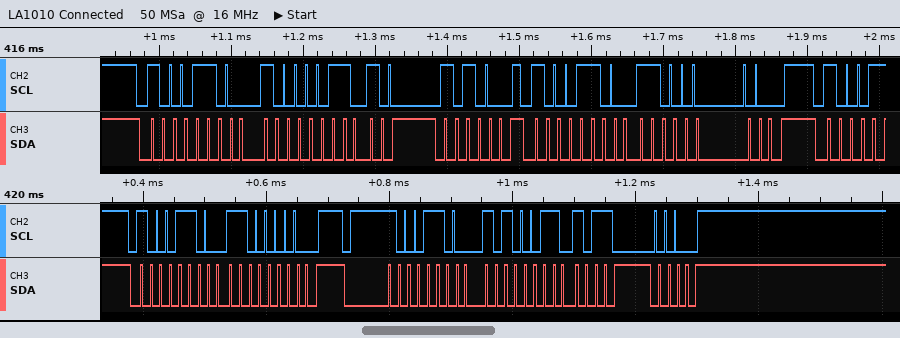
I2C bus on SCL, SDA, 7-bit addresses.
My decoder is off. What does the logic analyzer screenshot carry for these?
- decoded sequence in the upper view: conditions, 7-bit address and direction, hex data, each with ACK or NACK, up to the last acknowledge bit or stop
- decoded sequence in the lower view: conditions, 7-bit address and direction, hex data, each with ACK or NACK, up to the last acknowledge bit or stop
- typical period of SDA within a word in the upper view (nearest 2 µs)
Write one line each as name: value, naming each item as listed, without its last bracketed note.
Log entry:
decoded sequence in the upper view: conditions, 7-bit address and direction, hex data, each with ACK or NACK, up to the last acknowledge bit or stop: start, address 46 write ACK, 83 ACK, 94 ACK, stop, start, address 46 write ACK, C0 ACK, stop
decoded sequence in the lower view: conditions, 7-bit address and direction, hex data, each with ACK or NACK, up to the last acknowledge bit or stop: start, address 46 write ACK, C0 ACK, stop, start, address 46 write ACK, A3 ACK, B0 ACK, stop
typical period of SDA within a word in the upper view: 16 µs
